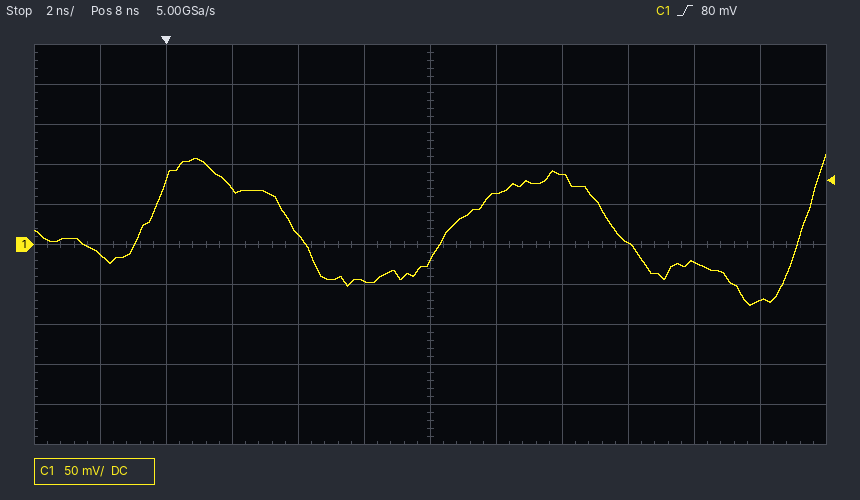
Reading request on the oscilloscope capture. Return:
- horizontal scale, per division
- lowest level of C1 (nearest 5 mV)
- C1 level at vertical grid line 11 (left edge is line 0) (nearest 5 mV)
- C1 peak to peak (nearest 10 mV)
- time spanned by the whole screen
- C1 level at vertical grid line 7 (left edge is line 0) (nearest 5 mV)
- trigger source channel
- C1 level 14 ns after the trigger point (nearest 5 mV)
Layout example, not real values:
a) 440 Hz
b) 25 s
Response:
a) 2 ns
b) -75 mV
c) -70 mV
d) 190 mV
e) 24 ns
f) 65 mV
g) C1
h) 0 mV
